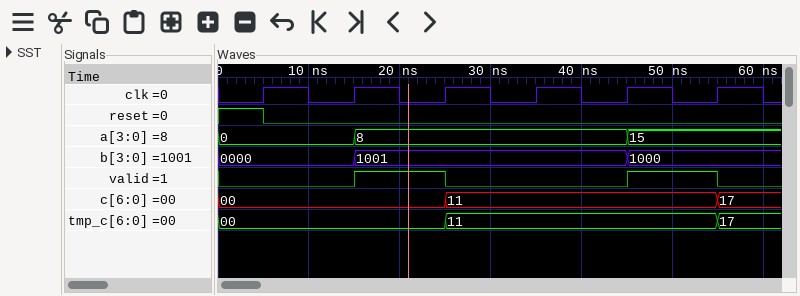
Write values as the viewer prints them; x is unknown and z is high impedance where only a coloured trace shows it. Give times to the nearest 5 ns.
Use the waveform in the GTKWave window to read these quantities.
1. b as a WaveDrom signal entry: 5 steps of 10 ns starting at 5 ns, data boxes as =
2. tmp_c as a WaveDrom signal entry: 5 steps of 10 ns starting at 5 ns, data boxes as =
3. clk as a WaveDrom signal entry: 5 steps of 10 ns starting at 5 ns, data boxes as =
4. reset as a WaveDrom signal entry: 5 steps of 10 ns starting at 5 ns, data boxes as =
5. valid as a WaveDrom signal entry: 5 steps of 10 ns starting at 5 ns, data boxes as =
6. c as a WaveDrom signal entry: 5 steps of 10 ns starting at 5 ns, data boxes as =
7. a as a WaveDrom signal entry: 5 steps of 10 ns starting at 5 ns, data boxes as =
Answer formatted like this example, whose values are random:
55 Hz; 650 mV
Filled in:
{name: 'b', wave: '==..=', data: '0000 1001 1000'}; {name: 'tmp_c', wave: '=.=..', data: '00 11'}; {name: 'clk', wave: 'p....'}; {name: 'reset', wave: '0....'}; {name: 'valid', wave: '010.1'}; {name: 'c', wave: '=.=..', data: '00 11'}; {name: 'a', wave: '==..=', data: '0 8 15'}
